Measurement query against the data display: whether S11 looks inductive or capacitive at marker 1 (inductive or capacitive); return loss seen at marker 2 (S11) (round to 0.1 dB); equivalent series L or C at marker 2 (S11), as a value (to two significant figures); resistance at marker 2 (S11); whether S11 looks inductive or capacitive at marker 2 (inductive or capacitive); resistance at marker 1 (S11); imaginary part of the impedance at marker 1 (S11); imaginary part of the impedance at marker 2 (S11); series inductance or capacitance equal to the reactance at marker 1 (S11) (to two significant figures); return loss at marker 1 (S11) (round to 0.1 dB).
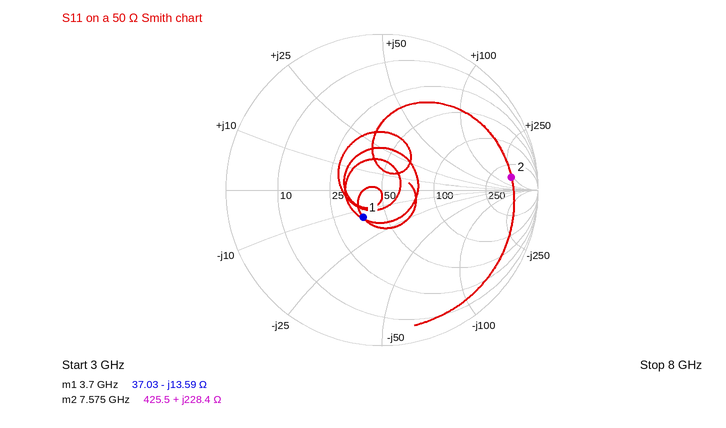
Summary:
capacitive
1.6 dB
4.8 nH
425.5 Ω
inductive
37.03 Ω
-13.59 Ω
+228.4 Ω
3.2 pF
13.4 dB
